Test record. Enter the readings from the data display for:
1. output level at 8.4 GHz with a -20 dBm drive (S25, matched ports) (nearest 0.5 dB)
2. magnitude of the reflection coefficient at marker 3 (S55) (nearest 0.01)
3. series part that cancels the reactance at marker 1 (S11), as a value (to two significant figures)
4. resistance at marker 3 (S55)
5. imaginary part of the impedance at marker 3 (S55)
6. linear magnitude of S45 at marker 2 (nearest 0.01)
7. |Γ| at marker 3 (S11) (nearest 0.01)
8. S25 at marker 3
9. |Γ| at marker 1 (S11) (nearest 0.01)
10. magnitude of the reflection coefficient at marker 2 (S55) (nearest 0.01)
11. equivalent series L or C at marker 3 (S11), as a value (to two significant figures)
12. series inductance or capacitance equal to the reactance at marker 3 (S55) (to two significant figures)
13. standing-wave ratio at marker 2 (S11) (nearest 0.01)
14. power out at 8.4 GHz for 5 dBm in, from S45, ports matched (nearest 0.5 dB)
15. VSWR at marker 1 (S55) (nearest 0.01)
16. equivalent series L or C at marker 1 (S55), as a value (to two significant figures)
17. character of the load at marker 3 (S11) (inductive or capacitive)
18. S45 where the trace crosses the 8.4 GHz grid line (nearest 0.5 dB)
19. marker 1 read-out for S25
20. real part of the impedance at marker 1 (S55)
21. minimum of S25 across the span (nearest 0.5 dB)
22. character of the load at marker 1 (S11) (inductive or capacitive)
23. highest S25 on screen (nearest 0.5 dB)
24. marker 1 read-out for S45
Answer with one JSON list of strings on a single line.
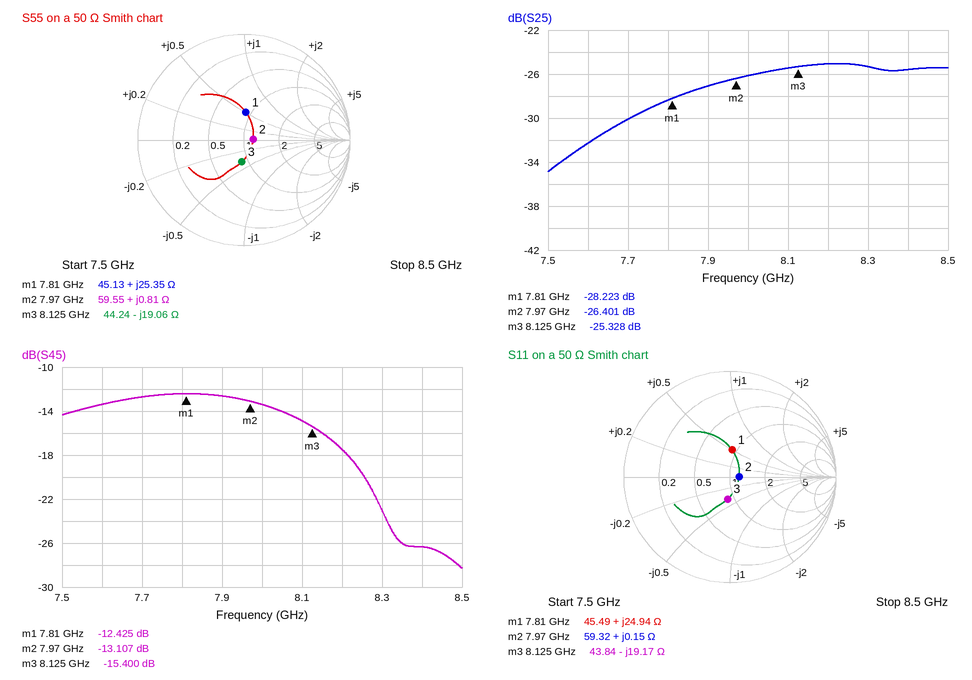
["-45.5 dBm", "0.21", "820 fF", "44.24 Ω", "-19.06 Ω", "0.22", "0.21", "-25.328 dB", "0.26", "0.09", "1.0 pF", "1.0 pF", "1.19", "-21.5 dBm", "1.71", "520 pH", "capacitive", "-26.5 dB", "-28.223 dB", "45.13 Ω", "-35.0 dB", "inductive", "-25.0 dB", "-12.425 dB"]
